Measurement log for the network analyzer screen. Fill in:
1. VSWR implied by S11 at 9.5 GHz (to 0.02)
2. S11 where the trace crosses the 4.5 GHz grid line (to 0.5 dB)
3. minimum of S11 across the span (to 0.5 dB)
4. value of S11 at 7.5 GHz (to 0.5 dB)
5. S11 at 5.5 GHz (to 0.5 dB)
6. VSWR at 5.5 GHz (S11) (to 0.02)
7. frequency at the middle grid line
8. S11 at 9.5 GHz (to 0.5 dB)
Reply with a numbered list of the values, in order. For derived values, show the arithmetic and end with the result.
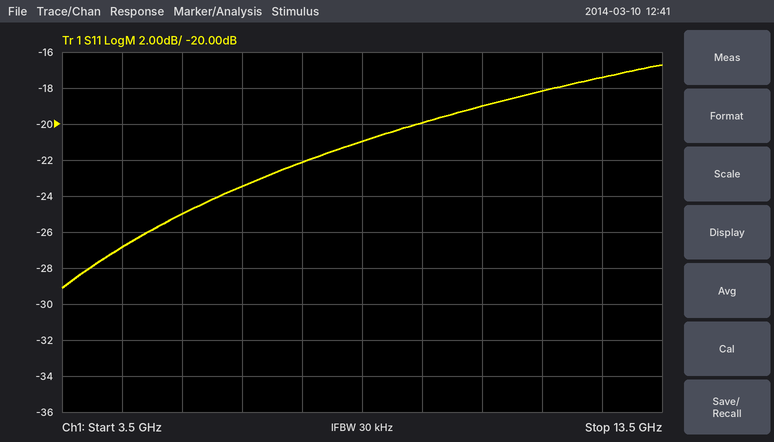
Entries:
1. |Γ| = 10^(-20/20) = 0.1000; VSWR = (1 + 0.1000)/(1 − 0.1000) ≈ 1.22
2. -27.0 dB
3. -29.0 dB
4. -22.0 dB
5. -25.0 dB
6. |Γ| = 10^(-25/20) = 0.0562; VSWR = (1 + 0.0562)/(1 − 0.0562) ≈ 1.12
7. 8.5 GHz
8. -20.0 dB
